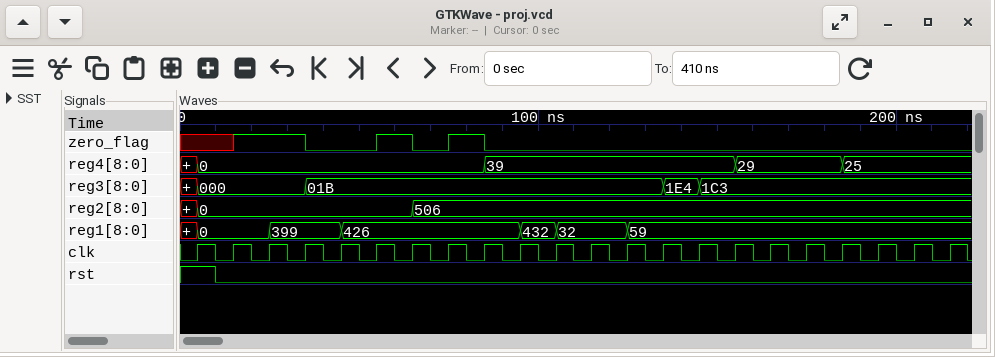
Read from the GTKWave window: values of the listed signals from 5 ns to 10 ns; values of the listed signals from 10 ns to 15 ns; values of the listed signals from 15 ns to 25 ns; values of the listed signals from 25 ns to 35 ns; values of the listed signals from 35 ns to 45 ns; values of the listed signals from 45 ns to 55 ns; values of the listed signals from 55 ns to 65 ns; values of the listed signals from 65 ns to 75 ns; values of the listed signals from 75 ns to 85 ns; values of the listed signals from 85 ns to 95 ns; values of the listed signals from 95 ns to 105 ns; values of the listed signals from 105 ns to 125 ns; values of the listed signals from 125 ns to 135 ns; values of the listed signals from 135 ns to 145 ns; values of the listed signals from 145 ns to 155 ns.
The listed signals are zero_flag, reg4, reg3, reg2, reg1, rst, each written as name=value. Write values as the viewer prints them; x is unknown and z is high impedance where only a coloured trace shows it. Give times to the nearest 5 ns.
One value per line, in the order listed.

zero_flag=x, reg4=0, reg3=000, reg2=0, reg1=0, rst=1
zero_flag=x, reg4=0, reg3=000, reg2=0, reg1=0, rst=0
zero_flag=1, reg4=0, reg3=000, reg2=0, reg1=0, rst=0
zero_flag=1, reg4=0, reg3=000, reg2=0, reg1=399, rst=0
zero_flag=0, reg4=0, reg3=01B, reg2=0, reg1=399, rst=0
zero_flag=0, reg4=0, reg3=01B, reg2=0, reg1=426, rst=0
zero_flag=1, reg4=0, reg3=01B, reg2=0, reg1=426, rst=0
zero_flag=0, reg4=0, reg3=01B, reg2=506, reg1=426, rst=0
zero_flag=1, reg4=0, reg3=01B, reg2=506, reg1=426, rst=0
zero_flag=0, reg4=39, reg3=01B, reg2=506, reg1=426, rst=0
zero_flag=0, reg4=39, reg3=01B, reg2=506, reg1=432, rst=0
zero_flag=0, reg4=39, reg3=01B, reg2=506, reg1=32, rst=0
zero_flag=0, reg4=39, reg3=01B, reg2=506, reg1=59, rst=0
zero_flag=0, reg4=39, reg3=1E4, reg2=506, reg1=59, rst=0
zero_flag=0, reg4=39, reg3=1C3, reg2=506, reg1=59, rst=0
